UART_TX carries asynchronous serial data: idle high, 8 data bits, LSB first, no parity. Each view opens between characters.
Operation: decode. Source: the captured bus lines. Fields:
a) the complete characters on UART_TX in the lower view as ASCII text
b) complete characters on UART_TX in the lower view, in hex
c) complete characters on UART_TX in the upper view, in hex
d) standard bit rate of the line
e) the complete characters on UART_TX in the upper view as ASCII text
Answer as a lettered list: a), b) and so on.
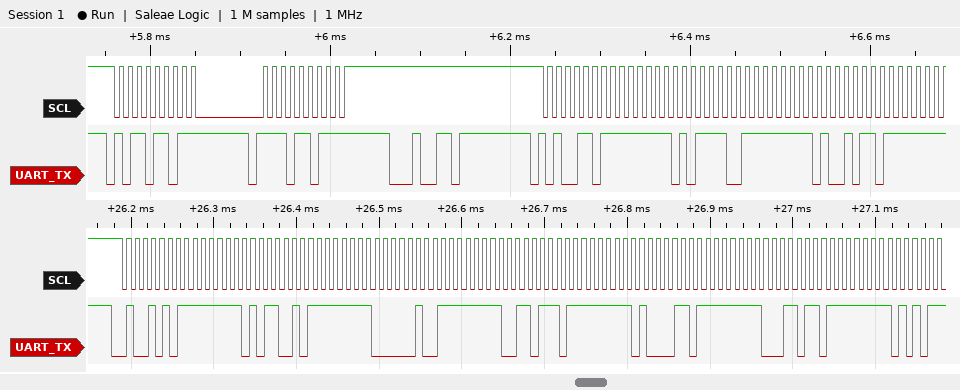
a) "RM val"
b) 52, 4D, 20, 76, 61, 6C
c) 6D, 6F, 64, 65, 3D, 69
d) 115200 baud
e) "mode=i"
